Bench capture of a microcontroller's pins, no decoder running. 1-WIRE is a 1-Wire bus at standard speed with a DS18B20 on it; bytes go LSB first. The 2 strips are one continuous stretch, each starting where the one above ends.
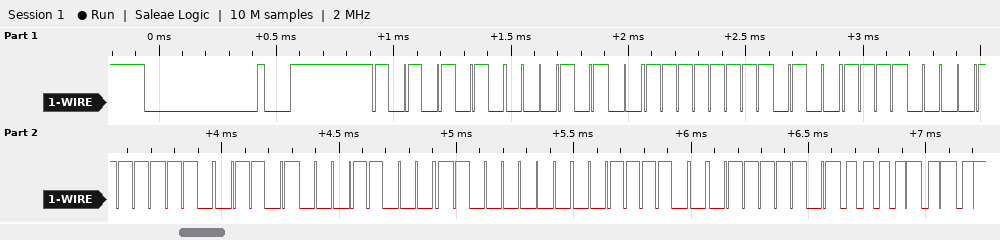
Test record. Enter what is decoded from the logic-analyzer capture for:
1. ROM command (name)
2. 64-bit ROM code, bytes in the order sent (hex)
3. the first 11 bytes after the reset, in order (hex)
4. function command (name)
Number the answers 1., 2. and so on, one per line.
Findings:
1. Match ROM
2. 28 FF F2 F0 B3 18 03 3C
3. 55 28 FF F2 F0 B3 18 03 3C BE 50
4. Read Scratchpad
